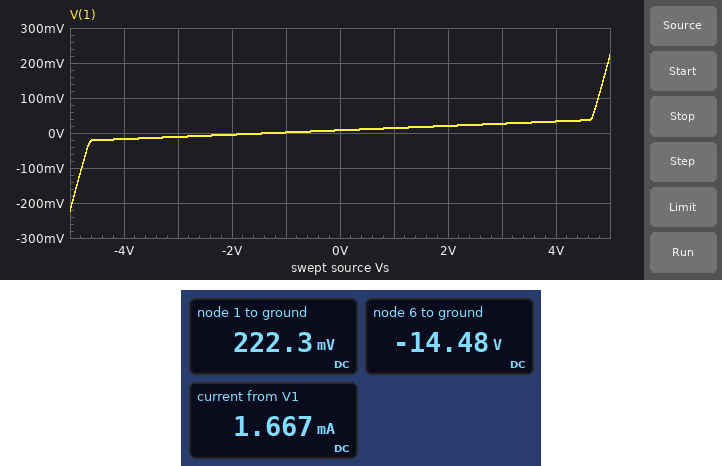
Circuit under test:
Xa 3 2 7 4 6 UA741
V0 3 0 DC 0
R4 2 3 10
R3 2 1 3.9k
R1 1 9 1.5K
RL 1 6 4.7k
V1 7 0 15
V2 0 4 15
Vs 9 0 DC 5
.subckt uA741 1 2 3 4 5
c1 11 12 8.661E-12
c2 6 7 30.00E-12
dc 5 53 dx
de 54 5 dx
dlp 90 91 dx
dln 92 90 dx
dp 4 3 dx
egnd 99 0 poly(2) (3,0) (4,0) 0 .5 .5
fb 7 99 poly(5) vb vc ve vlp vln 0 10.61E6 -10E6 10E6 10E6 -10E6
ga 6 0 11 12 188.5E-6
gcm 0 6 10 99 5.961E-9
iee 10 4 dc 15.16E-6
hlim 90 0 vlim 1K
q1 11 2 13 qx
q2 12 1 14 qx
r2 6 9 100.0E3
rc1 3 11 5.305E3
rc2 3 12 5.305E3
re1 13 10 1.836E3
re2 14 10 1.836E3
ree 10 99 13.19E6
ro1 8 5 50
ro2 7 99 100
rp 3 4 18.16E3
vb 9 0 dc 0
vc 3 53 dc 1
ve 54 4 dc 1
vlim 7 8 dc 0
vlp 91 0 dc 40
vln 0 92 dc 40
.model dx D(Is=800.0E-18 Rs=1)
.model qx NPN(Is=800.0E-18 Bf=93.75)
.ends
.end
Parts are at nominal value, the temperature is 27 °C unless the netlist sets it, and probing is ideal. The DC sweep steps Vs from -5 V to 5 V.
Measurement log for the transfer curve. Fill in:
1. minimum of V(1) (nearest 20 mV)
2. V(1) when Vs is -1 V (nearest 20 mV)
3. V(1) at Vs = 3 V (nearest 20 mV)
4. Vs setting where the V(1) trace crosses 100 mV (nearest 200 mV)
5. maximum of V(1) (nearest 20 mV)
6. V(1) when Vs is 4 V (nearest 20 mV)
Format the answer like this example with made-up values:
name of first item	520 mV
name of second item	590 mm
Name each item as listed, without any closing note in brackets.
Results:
minimum of V(1)	-220 mV
V(1) when Vs is -1 V	0 V
V(1) at Vs = 3 V	20 mV
Vs setting where the V(1) trace crosses 100 mV	4.8 V
maximum of V(1)	220 mV
V(1) when Vs is 4 V	40 mV
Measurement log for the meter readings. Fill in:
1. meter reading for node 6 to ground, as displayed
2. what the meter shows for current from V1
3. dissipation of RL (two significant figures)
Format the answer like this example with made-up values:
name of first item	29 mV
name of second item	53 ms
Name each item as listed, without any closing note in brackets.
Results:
meter reading for node 6 to ground, as displayed	-14.48 V
what the meter shows for current from V1	1.667 mA
dissipation of RL	46 mW
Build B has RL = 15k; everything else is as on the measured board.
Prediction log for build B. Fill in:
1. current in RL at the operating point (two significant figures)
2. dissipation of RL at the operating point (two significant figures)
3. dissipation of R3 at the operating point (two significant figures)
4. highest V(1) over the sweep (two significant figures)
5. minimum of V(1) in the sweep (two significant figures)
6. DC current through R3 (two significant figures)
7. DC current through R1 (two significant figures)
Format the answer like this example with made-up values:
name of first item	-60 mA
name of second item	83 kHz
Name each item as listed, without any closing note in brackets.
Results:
current in RL at the operating point	1.1 mA
dissipation of RL at the operating point	19 mW
dissipation of R3 at the operating point	1.5 mW
highest V(1) over the sweep	2.4 V
minimum of V(1) in the sweep	-2.4 V
DC current through R3	610 µA
DC current through R1	1.7 mA
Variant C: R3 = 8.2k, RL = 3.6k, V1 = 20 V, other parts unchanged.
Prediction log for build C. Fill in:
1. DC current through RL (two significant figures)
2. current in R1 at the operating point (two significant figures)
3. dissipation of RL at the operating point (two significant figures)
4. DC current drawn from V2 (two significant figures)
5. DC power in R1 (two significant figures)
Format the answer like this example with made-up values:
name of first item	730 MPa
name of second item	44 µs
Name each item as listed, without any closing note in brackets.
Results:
DC current through RL	3.2 mA
current in R1 at the operating point	3.2 mA
dissipation of RL at the operating point	37 mW
DC current drawn from V2	1.9 mA
DC power in R1	16 mW
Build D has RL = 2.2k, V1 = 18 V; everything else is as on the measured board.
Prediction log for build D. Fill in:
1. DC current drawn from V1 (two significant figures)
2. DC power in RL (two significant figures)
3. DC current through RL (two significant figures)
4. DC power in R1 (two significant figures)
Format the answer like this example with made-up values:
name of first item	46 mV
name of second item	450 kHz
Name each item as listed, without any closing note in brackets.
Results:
DC current drawn from V1	1.8 mA
DC power in RL	24 mW
DC current through RL	3.3 mA
DC power in R1	16 mW
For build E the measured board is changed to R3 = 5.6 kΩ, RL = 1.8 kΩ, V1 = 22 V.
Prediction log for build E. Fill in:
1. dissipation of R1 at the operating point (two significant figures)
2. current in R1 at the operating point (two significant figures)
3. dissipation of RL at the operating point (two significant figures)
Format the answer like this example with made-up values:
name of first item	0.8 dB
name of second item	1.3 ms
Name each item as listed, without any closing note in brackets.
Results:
dissipation of R1 at the operating point	16 mW
current in R1 at the operating point	3.3 mA
dissipation of RL at the operating point	19 mW
